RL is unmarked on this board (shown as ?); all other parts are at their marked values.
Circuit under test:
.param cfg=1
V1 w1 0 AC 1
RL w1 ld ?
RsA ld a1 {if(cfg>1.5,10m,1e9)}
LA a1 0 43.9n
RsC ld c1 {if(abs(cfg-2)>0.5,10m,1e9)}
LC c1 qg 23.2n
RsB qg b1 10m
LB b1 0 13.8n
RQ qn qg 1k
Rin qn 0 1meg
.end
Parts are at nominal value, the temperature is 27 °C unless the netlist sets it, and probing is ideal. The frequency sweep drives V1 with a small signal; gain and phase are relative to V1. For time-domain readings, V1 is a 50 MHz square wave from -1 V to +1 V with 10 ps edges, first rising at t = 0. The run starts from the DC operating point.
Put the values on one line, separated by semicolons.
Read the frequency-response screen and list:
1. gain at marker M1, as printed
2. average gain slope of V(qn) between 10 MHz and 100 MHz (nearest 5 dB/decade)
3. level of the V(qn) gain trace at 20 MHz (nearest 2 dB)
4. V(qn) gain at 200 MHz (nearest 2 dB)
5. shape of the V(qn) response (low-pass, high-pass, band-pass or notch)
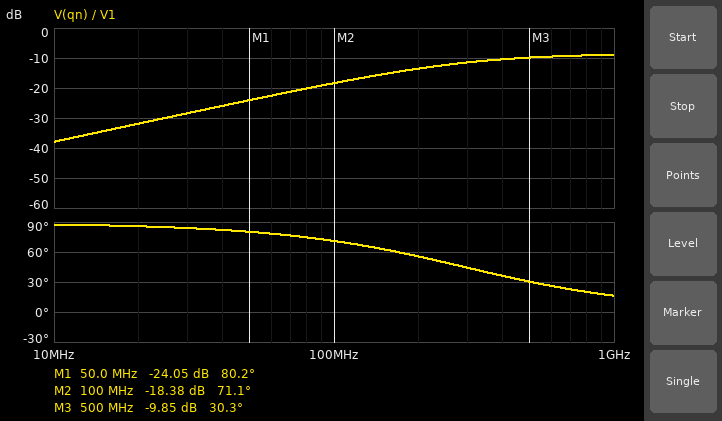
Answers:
-24.05 dB; 20 dB/decade; -32 dB; -14 dB; high-pass
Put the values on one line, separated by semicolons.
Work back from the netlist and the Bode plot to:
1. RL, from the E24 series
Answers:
68 Ω
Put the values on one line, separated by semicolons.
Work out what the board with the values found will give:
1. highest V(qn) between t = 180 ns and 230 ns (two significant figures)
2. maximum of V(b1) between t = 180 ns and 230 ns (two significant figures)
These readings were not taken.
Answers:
740 mV; 740 mV
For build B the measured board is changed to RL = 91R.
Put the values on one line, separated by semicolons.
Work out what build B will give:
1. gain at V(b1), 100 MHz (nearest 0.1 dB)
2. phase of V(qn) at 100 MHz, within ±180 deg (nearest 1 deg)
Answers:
-20.7 dB; 76 deg
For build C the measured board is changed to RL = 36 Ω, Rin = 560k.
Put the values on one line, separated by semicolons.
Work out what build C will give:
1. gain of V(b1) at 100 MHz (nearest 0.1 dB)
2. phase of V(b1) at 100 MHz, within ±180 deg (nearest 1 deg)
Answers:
-13.9 dB; 57 deg
